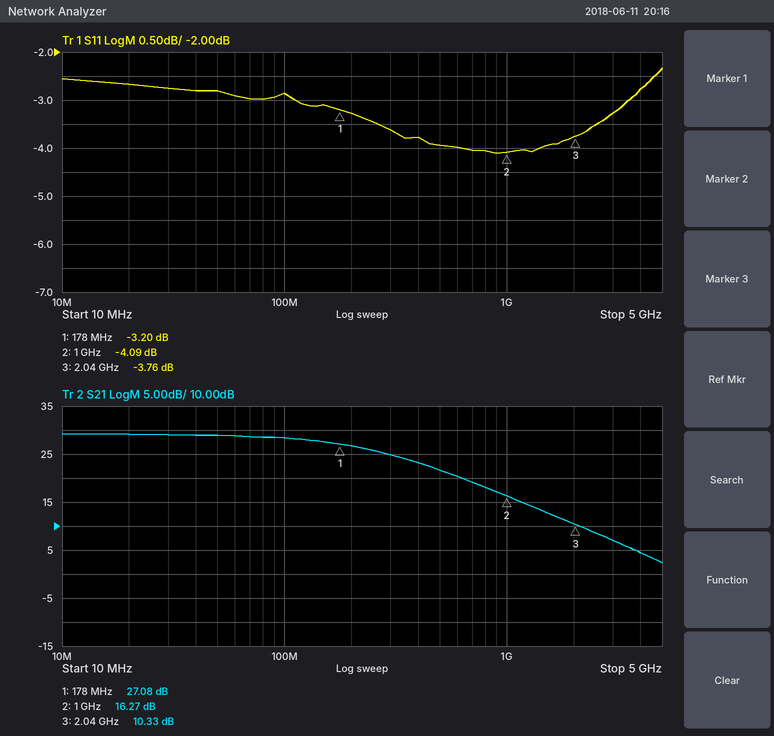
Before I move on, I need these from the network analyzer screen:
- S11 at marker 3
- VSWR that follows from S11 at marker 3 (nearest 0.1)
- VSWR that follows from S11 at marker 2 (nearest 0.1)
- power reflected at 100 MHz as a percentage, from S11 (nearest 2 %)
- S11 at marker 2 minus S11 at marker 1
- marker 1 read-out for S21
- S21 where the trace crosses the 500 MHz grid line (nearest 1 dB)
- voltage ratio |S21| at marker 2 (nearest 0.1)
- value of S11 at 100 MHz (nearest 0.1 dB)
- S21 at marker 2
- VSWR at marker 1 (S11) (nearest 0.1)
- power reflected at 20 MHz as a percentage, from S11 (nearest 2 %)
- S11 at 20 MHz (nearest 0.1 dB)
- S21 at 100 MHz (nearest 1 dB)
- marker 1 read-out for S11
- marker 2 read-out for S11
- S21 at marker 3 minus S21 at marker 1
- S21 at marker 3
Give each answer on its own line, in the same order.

-3.76 dB
4.7
4.3
52 %
-0.89 dB
27.08 dB
22 dB
6.5
-2.9 dB
16.27 dB
5.5
54 %
-2.7 dB
28 dB
-3.20 dB
-4.09 dB
-16.75 dB
10.33 dB
